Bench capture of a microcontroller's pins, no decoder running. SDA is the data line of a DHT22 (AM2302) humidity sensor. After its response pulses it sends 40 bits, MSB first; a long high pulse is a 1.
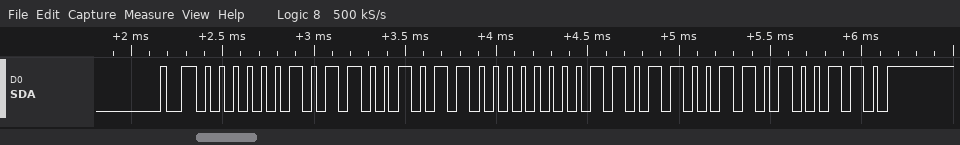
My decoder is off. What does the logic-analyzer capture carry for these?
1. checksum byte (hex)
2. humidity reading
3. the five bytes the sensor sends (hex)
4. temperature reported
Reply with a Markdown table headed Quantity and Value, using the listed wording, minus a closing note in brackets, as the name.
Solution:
| Quantity | Value |
|---|---|
| checksum byte | 0xA6 |
| humidity reading | 71.5 % |
| the five bytes the sensor sends | 02 CB 00 D9 A6 |
| temperature reported | 21.7 °C |
